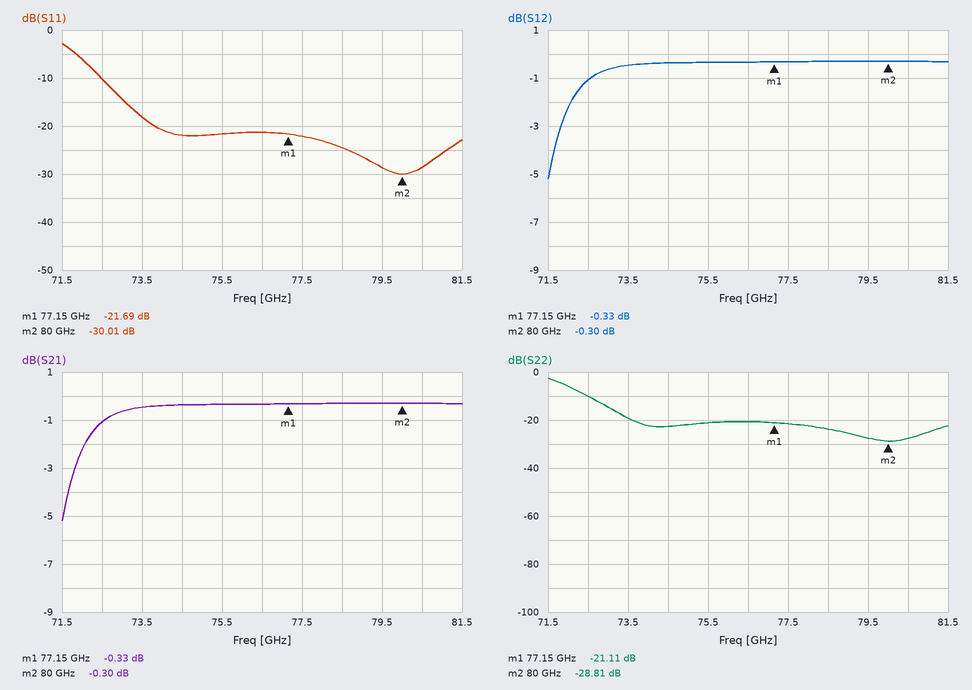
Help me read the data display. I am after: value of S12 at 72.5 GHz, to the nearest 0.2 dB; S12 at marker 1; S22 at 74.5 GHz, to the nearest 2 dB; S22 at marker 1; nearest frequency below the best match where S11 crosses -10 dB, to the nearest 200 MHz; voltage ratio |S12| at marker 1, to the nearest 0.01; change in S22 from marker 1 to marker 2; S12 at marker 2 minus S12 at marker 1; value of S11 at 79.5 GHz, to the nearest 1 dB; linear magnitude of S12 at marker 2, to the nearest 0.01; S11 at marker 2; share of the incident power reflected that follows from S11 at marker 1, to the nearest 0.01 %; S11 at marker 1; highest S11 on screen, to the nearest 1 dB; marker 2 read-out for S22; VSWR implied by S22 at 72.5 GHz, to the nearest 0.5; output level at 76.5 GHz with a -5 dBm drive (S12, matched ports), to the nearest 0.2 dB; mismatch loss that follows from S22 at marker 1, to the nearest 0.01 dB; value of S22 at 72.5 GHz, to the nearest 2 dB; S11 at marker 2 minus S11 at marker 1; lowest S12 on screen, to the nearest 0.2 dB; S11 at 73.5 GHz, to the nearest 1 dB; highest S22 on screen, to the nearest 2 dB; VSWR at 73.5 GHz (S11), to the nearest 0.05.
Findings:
-1.0 dB
-0.33 dB
-22 dB
-21.11 dB
72.4 GHz
0.96
-7.70 dB
0.03 dB
-29 dB
0.97
-30.01 dB
0.68 %
-21.69 dB
-3 dB
-28.81 dB
2.0
-5.4 dBm
0.03 dB
-10 dB
-8.32 dB
-5.2 dB
-18 dB
-2 dB
1.30
